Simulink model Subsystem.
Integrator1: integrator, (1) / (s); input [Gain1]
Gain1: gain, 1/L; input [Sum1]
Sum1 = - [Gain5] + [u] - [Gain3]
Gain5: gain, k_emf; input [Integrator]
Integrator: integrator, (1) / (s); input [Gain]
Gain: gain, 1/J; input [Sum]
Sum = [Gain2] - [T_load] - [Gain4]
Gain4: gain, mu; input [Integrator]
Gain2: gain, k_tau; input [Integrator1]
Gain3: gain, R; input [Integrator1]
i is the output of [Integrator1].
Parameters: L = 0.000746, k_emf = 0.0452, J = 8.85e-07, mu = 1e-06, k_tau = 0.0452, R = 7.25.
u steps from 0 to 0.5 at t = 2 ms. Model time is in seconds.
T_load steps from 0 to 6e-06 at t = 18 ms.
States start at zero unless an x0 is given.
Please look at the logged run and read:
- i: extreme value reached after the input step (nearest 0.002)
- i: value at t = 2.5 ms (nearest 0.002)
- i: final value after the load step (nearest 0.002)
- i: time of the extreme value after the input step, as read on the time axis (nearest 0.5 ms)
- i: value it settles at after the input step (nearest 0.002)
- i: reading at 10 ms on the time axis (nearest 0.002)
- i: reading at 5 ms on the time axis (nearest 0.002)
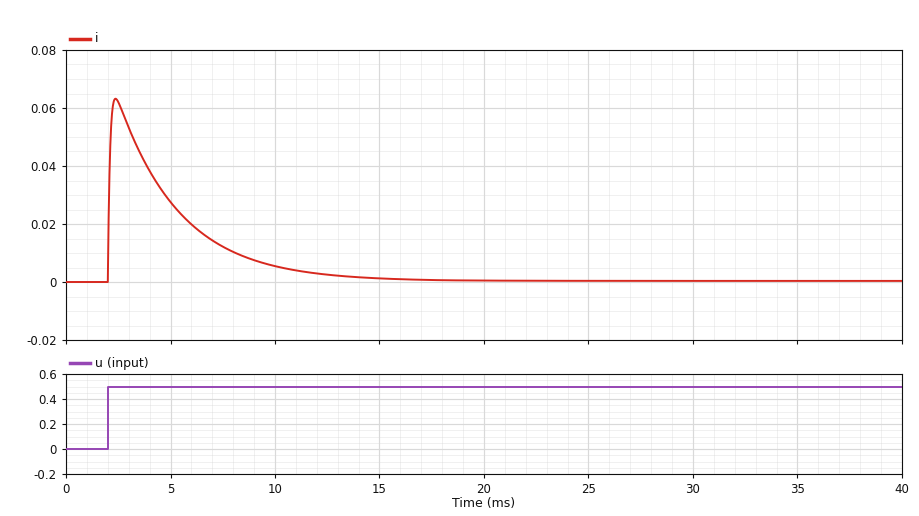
0.064
0.062
0.000
2.5 ms
0.000
0.006
0.028
